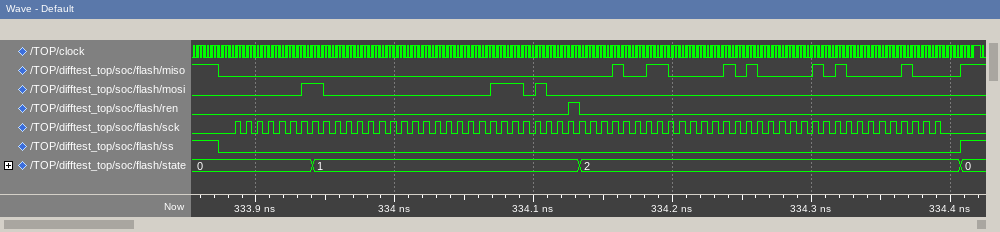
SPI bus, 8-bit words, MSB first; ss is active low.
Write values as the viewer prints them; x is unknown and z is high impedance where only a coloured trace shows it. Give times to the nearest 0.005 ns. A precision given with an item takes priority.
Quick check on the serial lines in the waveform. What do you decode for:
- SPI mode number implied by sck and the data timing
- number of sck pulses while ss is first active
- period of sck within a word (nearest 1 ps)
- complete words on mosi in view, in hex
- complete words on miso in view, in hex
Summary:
1
64
8 ps
03, 00, 01, D0, 00, 00, 00, 00
00, 00, 00, 00, 26, 0A, 0A, 08
